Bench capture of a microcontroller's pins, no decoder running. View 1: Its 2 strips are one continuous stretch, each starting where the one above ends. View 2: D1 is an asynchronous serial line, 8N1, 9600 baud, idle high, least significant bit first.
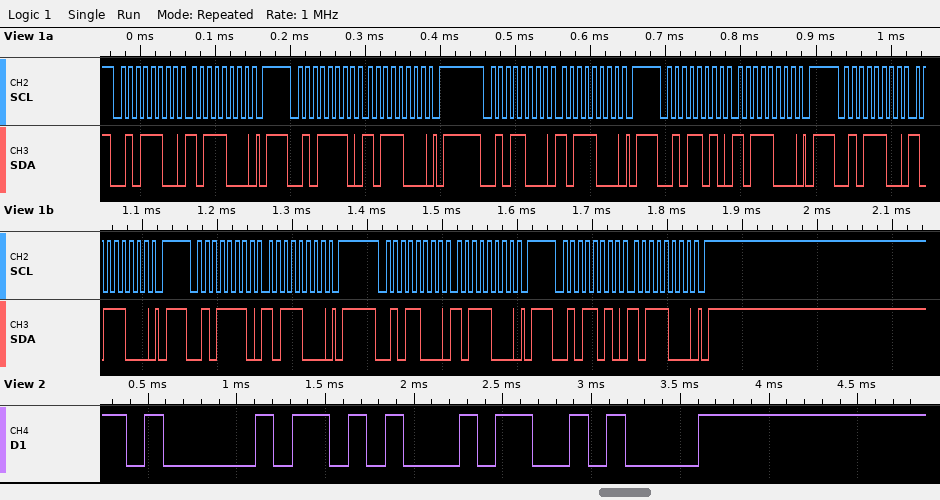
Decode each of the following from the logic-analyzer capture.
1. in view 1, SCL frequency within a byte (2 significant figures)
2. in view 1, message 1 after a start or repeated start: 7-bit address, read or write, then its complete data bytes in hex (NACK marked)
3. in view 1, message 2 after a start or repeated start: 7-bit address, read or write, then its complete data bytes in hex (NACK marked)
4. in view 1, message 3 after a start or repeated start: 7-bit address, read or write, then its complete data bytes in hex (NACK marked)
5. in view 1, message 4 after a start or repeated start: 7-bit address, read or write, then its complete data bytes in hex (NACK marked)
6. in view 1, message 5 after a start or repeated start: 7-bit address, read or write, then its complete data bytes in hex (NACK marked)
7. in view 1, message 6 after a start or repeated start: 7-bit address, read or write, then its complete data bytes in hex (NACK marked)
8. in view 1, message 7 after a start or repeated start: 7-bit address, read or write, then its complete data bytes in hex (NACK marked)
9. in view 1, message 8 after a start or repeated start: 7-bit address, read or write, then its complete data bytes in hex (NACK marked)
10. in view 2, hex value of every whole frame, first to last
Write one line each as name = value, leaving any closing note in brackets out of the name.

in view 1, SCL frequency within a byte = 100 kHz
in view 1, message 1 after a start or repeated start: 7-bit address, read or write, then its complete data bytes in hex = 0x2E write: B8
in view 1, message 2 after a start or repeated start: 7-bit address, read or write, then its complete data bytes in hex = 0x2F write: B8
in view 1, message 3 after a start or repeated start: 7-bit address, read or write, then its complete data bytes in hex = 0x2C write: B8
in view 1, message 4 after a start or repeated start: 7-bit address, read or write, then its complete data bytes in hex = 0x2D write: B8
in view 1, message 5 after a start or repeated start: 7-bit address, read or write, then its complete data bytes in hex = 0x2E write: B8
in view 1, message 6 after a start or repeated start: 7-bit address, read or write, then its complete data bytes in hex = 0x2F write: B8
in view 1, message 7 after a start or repeated start: 7-bit address, read or write, then its complete data bytes in hex = 0x2C write: B8
in view 1, message 8 after a start or repeated start: 7-bit address, read or write, then its complete data bytes in hex = 0x2D write: B8
in view 2, hex value of every whole frame, first to last = 0x41 0x45 0x0A
